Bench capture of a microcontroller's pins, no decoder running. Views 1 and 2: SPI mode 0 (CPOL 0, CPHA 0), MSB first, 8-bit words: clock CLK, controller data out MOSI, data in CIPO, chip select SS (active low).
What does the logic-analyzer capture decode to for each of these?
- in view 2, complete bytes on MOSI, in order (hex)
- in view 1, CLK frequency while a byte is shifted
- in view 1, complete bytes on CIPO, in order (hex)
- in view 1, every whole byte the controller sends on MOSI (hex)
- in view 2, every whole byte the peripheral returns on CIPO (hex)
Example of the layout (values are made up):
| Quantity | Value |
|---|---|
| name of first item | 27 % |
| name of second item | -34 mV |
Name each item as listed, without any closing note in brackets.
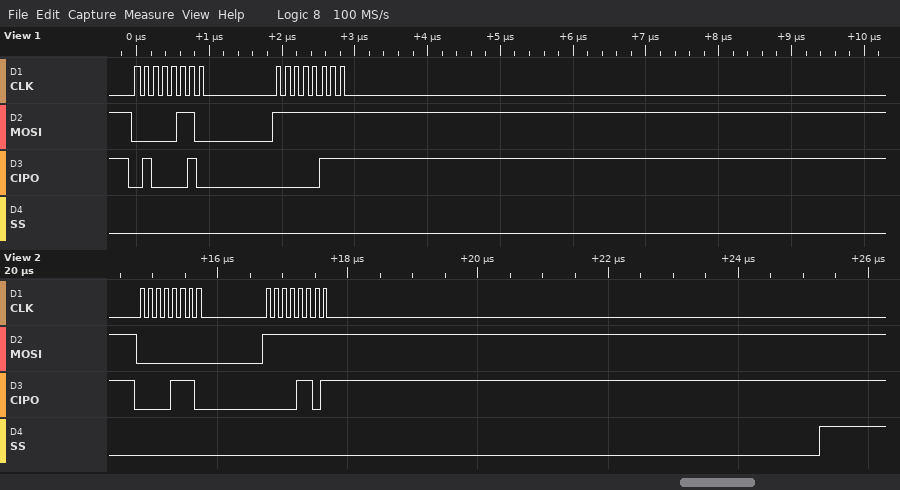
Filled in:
| Quantity | Value |
|---|---|
| in view 2, complete bytes on MOSI, in order | 00 FF |
| in view 1, CLK frequency while a byte is shifted | 8 MHz |
| in view 1, complete bytes on CIPO, in order | 0x42 0x07 |
| in view 1, every whole byte the controller sends on MOSI | 0x06 0xFF |
| in view 2, every whole byte the peripheral returns on CIPO | 0E 0D |
